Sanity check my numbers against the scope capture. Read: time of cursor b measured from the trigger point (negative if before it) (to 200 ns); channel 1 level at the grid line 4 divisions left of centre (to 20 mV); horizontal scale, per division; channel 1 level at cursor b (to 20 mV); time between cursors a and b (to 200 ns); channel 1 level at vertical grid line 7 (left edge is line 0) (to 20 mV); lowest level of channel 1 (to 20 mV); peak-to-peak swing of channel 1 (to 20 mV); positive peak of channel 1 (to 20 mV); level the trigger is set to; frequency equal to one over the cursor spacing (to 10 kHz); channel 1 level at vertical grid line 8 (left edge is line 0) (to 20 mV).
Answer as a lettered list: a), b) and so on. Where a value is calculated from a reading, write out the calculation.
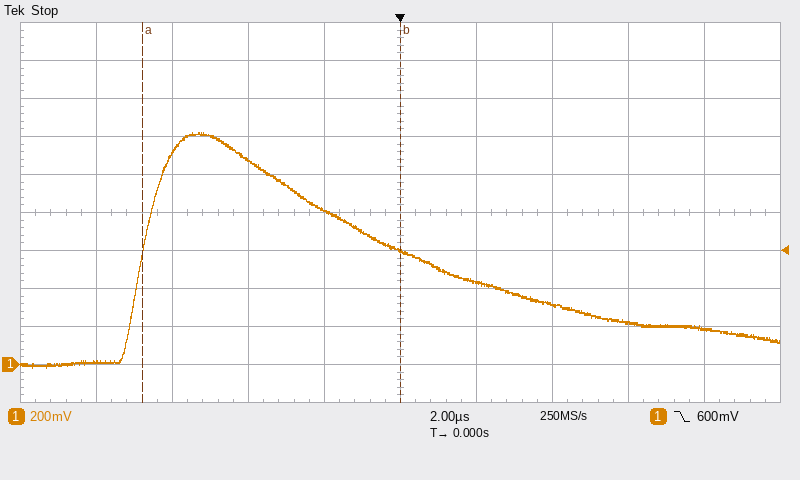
a) 0.0 µs
b) 20 mV
c) 2 µs
d) 600 mV
e) 6.8 µs
f) 320 mV
g) -20 mV
h) 1.22 V − (-20 mV) = 1.24 V
i) 1.22 V
j) 600 mV
k) 1 / 6.8 µs ≈ 150 kHz
l) 220 mV
